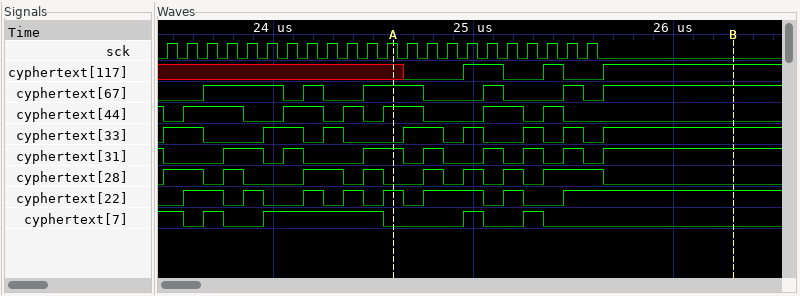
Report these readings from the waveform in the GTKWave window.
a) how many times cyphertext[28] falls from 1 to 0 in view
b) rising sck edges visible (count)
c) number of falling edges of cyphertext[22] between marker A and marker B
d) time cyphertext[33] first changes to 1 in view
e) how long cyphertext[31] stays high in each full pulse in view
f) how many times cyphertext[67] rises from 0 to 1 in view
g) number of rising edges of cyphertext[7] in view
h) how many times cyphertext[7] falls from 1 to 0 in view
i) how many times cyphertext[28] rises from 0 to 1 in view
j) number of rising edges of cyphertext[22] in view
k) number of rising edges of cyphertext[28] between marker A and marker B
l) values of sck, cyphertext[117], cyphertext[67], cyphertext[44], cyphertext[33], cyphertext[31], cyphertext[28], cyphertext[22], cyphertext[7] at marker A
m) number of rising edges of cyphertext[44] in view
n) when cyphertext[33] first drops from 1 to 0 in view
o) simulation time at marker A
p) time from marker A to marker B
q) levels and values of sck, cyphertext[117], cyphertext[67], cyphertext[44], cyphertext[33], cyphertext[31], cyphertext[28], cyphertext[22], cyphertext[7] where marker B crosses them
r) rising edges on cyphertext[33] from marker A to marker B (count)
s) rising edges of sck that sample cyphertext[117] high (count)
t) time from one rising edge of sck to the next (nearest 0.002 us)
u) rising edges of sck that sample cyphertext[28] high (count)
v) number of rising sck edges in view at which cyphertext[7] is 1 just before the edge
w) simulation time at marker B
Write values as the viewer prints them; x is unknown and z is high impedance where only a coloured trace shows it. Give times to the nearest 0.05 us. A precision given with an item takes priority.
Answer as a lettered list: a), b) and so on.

a) 8
b) 22
c) 3
d) 23.45 us
e) 0.2 us, 0.1 us, 0.2 us, 0.1 us, 0.1 us, 0.1 us, 0.1 us
f) 6
g) 4
h) 5
i) 8
j) 8
k) 4
l) sck=1, cyphertext[117]=x, cyphertext[67]=1, cyphertext[44]=1, cyphertext[33]=0, cyphertext[31]=1, cyphertext[28]=0, cyphertext[22]=1, cyphertext[7]=0
m) 6
n) 23.65 us
o) 24.6 us
p) 1.7 us
q) sck=0, cyphertext[117]=1, cyphertext[67]=1, cyphertext[44]=0, cyphertext[33]=1, cyphertext[31]=1, cyphertext[28]=0, cyphertext[22]=1, cyphertext[7]=0
r) 5
s) 3
t) 0.1 us
u) 12
v) 10
w) 26.3 us
